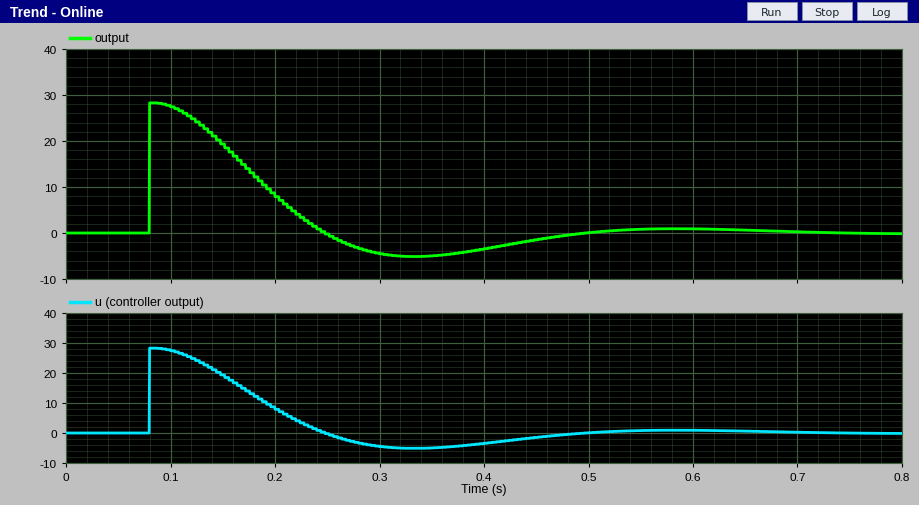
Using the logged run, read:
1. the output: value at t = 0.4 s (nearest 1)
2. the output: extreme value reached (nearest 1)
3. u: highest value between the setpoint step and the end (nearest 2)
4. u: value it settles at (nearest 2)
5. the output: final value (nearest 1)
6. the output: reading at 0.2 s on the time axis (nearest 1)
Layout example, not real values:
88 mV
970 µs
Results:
-3
28
28
0
0
8
